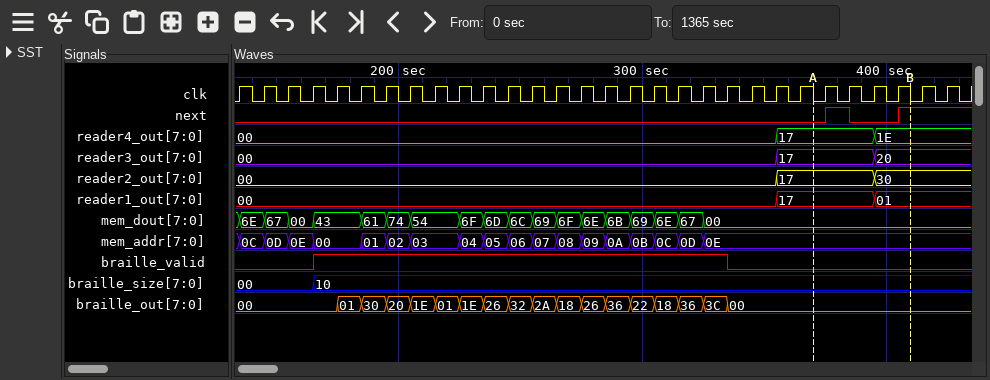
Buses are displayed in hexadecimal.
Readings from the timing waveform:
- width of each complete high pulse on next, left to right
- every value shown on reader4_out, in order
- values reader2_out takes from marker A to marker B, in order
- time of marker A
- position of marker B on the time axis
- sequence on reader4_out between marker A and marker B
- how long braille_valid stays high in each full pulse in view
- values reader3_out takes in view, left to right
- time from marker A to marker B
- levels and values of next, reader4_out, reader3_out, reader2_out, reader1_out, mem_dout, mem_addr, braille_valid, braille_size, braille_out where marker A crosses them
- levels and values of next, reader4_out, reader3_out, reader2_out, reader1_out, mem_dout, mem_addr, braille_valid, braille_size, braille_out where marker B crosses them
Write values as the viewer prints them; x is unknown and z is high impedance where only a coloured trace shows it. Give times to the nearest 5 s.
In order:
10 s
00, 17, 1E
17, 30
370 s
410 s
17, 1E
170 s
00, 17, 20
40 s
next=0, reader4_out=17, reader3_out=17, reader2_out=17, reader1_out=17, mem_dout=00, mem_addr=0E, braille_valid=0, braille_size=10, braille_out=00
next=1, reader4_out=1E, reader3_out=20, reader2_out=30, reader1_out=01, mem_dout=00, mem_addr=0E, braille_valid=0, braille_size=10, braille_out=00
